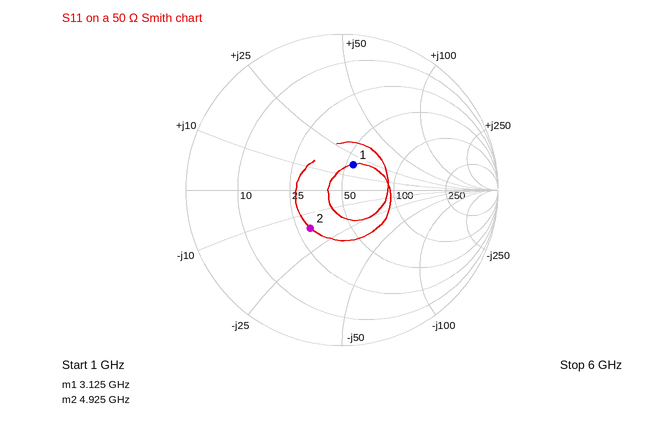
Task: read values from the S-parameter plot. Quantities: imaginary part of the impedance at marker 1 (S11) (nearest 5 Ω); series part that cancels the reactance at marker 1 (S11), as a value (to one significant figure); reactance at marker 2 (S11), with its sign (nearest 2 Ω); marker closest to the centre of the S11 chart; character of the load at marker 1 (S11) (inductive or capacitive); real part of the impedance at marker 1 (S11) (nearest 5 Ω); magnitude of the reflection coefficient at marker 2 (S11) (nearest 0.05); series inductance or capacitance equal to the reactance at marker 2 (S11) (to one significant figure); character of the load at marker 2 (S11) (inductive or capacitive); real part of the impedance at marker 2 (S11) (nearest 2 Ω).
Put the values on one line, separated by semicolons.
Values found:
+20 Ω; 3 pF; -16 Ω; marker 1; inductive; 55 Ω; 0.30; 2 pF; capacitive; 30 Ω
